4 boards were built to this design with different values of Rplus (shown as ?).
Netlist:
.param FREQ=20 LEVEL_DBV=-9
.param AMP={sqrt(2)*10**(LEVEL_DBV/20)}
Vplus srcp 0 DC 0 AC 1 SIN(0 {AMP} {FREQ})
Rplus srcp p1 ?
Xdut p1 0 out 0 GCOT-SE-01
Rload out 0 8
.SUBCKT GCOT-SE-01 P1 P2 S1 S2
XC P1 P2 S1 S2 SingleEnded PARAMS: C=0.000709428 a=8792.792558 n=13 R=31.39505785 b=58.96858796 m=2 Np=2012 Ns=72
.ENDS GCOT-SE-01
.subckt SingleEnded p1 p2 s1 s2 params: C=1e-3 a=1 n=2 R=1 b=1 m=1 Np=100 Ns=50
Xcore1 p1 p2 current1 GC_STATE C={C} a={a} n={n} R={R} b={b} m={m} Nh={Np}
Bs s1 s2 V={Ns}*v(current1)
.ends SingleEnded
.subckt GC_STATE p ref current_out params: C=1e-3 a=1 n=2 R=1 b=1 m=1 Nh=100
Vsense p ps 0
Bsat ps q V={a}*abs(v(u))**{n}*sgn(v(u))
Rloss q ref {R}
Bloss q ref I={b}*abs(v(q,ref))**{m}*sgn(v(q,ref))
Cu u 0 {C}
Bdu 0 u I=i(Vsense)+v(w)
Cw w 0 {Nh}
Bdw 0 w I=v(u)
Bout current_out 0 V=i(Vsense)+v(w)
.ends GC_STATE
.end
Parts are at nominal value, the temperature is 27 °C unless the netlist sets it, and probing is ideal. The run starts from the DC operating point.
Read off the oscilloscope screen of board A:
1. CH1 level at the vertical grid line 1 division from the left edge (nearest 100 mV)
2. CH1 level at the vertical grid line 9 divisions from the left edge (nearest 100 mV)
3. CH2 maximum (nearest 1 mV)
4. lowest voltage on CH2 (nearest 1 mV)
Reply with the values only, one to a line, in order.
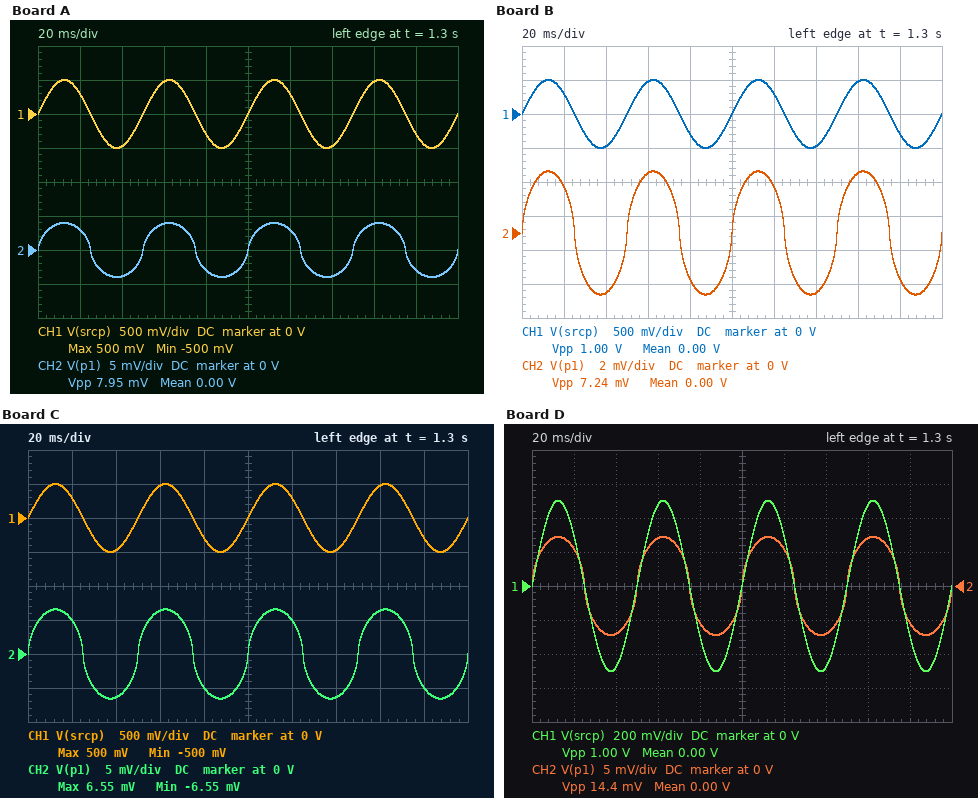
300 mV
-300 mV
4 mV
-4 mV
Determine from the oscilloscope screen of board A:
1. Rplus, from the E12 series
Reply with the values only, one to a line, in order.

470 Ω
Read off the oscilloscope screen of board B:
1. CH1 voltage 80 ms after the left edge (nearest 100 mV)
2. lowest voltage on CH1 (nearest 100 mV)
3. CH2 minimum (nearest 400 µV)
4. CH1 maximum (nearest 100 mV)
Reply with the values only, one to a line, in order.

-300 mV
-500 mV
-3.6 mV
500 mV
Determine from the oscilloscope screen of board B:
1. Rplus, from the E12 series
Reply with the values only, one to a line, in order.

560 Ω
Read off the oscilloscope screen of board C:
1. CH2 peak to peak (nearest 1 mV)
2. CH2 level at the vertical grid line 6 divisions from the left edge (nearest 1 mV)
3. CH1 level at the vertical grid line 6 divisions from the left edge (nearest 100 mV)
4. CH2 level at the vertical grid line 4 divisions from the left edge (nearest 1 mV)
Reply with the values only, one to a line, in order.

13 mV
5 mV
300 mV
-5 mV
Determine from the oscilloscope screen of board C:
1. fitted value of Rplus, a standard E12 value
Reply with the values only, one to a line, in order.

180 Ω
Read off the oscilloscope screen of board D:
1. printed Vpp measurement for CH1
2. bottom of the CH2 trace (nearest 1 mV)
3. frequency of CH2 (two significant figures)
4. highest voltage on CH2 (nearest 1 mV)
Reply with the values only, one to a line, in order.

1.00 V
-7 mV
20 Hz
7 mV
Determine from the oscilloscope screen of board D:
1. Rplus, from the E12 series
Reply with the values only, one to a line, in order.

150 Ω
